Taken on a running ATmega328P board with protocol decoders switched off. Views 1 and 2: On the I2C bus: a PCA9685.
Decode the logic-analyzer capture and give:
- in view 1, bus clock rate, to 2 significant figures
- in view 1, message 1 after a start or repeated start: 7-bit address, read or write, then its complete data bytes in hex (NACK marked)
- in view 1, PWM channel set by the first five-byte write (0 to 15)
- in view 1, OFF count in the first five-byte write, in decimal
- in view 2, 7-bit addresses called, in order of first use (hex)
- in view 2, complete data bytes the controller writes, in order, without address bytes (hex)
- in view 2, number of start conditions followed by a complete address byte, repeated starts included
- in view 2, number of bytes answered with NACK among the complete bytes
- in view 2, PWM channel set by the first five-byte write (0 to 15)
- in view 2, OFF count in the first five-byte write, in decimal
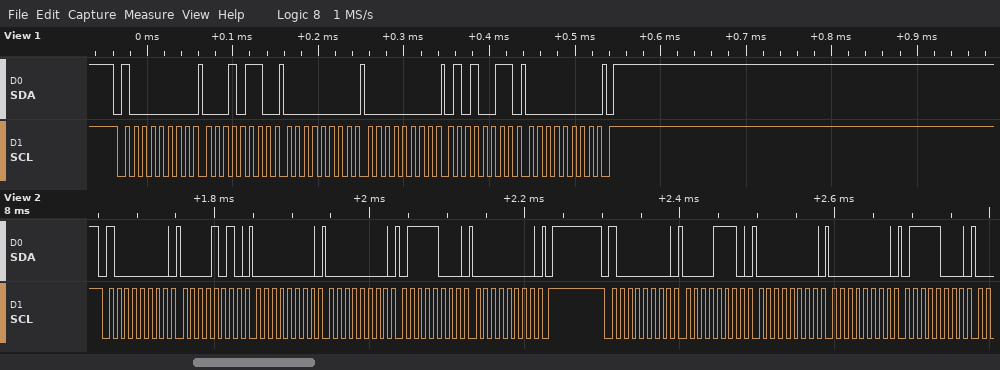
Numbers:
100 kHz
0x40 write: 16 00 00 53 00
4
83
0x40
0A 00 00 78 00 0E 00 00 78
2
0
1
120
